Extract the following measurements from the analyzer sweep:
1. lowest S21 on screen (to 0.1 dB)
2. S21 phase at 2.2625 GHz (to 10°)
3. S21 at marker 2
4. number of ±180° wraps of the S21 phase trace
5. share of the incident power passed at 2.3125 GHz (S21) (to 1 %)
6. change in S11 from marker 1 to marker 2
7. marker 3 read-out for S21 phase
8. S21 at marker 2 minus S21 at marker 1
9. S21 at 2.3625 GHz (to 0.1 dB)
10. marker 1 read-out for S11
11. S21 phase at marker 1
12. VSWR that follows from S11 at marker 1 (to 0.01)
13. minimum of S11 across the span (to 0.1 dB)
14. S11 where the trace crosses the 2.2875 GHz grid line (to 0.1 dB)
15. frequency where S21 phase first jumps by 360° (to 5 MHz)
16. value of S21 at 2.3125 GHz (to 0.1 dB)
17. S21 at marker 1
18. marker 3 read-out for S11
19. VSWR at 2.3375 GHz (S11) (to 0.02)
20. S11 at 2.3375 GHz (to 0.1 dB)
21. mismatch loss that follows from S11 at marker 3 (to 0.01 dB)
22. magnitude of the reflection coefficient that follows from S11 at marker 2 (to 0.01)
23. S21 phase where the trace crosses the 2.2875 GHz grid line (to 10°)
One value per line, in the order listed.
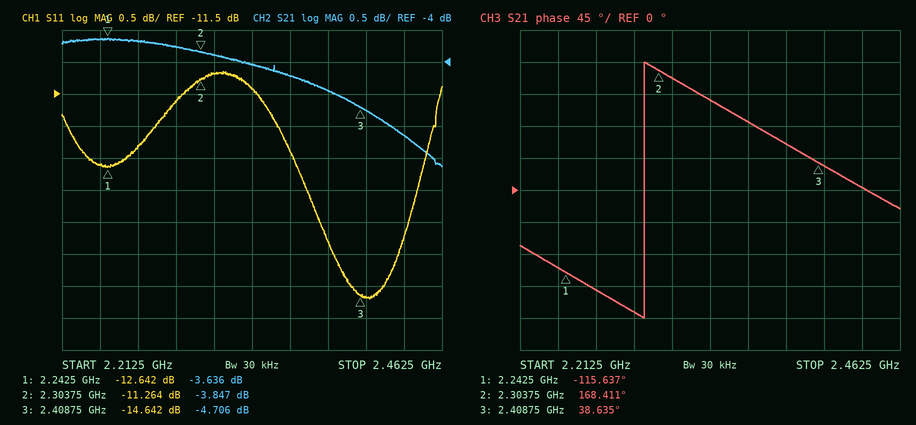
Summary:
-5.6 dB
-140°
-3.847 dB
1
41 %
1.378 dB
38.635°
-0.211 dB
-4.2 dB
-12.642 dB
-115.637°
1.61
-14.7 dB
-11.6 dB
2.295 GHz
-3.9 dB
-3.636 dB
-14.642 dB
1.74
-11.4 dB
0.15 dB
0.27
-170°
